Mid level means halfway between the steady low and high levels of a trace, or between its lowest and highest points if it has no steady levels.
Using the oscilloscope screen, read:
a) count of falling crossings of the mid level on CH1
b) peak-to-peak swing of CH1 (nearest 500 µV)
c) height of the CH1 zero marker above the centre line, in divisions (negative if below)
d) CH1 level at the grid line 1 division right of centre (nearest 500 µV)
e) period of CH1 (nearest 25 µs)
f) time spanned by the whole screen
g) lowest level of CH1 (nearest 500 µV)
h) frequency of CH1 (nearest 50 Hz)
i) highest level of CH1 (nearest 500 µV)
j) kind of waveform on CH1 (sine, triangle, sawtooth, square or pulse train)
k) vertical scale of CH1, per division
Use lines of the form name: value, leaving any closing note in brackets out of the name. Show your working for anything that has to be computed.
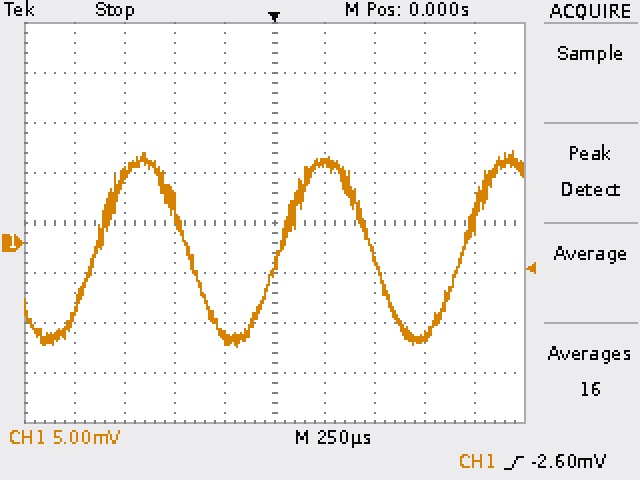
count of falling crossings of the mid level on CH1: 2
peak-to-peak swing of CH1: 9.0 mV − (-10.5 mV) = 19.5 mV
height of the CH1 zero marker above the centre line, in divisions: -0.4 div
CH1 level at the grid line 1 division right of centre: 8.0 mV
period of CH1: 925 µs
time spanned by the whole screen: 2.5 ms
lowest level of CH1: -10.5 mV
frequency of CH1: 1 / 925 µs ≈ 1.08 kHz, so 1.10 kHz to the nearest 50 Hz
highest level of CH1: 9.0 mV
kind of waveform on CH1: sine
vertical scale of CH1, per division: 5 mV
